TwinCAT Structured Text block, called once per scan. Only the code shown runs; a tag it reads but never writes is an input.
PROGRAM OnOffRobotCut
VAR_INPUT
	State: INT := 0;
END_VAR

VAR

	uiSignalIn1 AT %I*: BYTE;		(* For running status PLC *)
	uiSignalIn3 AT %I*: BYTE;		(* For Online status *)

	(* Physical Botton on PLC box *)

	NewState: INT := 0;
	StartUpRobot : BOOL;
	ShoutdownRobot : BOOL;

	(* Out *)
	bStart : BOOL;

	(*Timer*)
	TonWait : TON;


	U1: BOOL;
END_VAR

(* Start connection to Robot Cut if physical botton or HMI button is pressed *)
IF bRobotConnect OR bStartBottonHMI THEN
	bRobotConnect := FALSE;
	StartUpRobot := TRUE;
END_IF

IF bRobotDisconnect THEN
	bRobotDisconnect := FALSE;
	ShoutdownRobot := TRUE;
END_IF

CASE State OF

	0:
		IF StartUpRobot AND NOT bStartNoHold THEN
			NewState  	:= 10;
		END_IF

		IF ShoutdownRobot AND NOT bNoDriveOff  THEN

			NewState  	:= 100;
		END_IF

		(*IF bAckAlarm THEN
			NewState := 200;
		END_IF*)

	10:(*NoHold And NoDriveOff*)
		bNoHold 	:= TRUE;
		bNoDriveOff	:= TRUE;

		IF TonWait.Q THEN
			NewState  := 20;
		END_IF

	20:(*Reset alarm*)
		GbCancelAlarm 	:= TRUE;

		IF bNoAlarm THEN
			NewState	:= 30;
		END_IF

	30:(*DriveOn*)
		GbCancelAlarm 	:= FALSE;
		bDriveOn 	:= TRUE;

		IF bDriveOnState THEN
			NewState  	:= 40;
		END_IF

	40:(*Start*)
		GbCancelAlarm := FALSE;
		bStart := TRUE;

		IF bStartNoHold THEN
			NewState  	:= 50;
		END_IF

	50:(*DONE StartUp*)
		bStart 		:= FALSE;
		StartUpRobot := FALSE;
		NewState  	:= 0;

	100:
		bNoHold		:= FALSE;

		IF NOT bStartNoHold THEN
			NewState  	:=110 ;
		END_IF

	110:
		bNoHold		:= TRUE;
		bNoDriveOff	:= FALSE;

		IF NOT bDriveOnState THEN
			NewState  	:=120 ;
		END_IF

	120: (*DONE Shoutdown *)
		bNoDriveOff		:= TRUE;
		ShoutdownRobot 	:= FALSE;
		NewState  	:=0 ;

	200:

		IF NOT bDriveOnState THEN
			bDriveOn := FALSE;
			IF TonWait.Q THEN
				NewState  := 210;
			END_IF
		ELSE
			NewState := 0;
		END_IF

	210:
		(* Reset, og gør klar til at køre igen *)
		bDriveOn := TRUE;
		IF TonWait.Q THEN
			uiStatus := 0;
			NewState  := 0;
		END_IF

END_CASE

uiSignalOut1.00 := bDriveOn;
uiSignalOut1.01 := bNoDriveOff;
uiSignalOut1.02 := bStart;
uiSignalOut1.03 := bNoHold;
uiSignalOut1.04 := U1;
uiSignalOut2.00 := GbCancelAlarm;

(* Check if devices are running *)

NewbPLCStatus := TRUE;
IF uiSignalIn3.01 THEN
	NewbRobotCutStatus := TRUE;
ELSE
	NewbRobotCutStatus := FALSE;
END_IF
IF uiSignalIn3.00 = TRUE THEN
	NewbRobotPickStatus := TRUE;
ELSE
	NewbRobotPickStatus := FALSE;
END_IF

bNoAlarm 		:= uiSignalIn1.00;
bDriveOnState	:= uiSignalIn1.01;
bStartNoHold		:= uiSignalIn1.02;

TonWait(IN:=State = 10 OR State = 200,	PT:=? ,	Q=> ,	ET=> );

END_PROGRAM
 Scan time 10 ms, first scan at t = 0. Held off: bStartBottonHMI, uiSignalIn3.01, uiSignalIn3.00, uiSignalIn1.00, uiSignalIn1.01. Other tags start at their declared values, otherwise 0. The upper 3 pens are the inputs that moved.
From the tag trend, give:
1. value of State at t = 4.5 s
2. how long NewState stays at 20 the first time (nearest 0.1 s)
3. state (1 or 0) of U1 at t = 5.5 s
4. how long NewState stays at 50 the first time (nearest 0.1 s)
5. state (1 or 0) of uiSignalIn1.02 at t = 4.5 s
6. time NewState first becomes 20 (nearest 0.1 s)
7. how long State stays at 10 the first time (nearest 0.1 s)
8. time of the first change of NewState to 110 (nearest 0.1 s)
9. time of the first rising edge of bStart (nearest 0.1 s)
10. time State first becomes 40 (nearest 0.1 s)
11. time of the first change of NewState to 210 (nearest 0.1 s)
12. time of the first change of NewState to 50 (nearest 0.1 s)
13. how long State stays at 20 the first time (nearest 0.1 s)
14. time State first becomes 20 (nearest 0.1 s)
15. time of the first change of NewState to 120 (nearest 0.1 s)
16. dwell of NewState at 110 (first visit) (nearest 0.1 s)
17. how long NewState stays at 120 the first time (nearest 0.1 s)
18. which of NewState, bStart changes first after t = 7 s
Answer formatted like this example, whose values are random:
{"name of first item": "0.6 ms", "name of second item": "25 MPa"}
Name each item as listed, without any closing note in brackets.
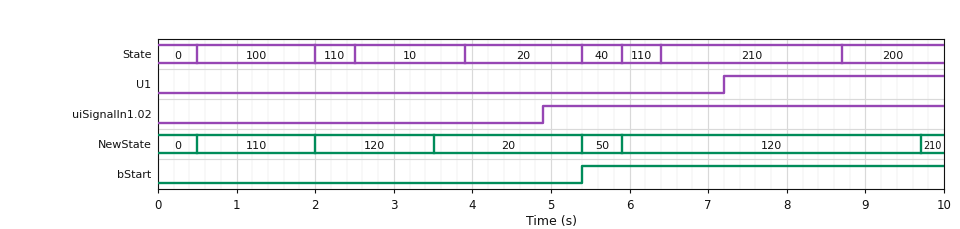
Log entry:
{"value of State at t = 4.5 s": "20", "how long NewState stays at 20 the first time": "1.9 s", "state (1 or 0) of U1 at t = 5.5 s": "0", "how long NewState stays at 50 the first time": "0.5 s", "state (1 or 0) of uiSignalIn1.02 at t = 4.5 s": "0", "time NewState first becomes 20": "3.5 s", "how long State stays at 10 the first time": "1.4 s", "time of the first change of NewState to 110": "0.5 s", "time of the first rising edge of bStart": "5.4 s", "time State first becomes 40": "5.4 s", "time of the first change of NewState to 210": "9.7 s", "time of the first change of NewState to 50": "5.4 s", "how long State stays at 20 the first time": "1.5 s", "time State first becomes 20": "3.9 s", "time of the first change of NewState to 120": "2.0 s", "dwell of NewState at 110 (first visit)": "1.5 s", "how long NewState stays at 120 the first time": "1.5 s", "which of NewState, bStart changes first after t = 7 s": "NewState"}
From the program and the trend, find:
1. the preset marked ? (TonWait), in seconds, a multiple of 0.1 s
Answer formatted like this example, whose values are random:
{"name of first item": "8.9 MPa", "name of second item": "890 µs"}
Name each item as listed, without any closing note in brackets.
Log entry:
{"the preset marked ? (TonWait), in seconds, a multiple of 0.1 s": "1.0 s"}
